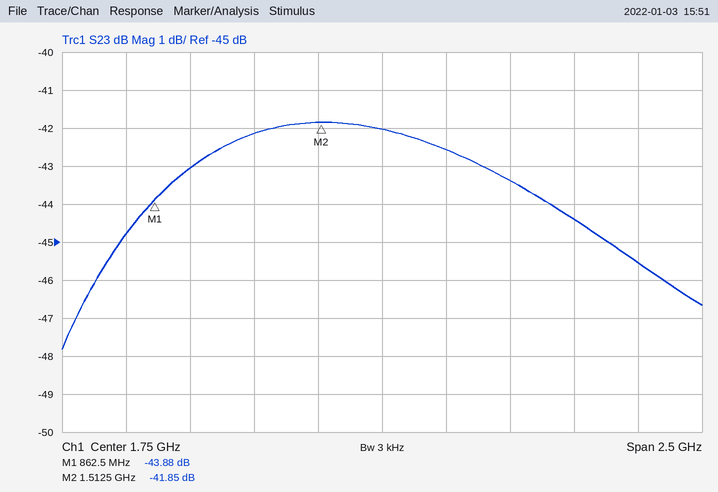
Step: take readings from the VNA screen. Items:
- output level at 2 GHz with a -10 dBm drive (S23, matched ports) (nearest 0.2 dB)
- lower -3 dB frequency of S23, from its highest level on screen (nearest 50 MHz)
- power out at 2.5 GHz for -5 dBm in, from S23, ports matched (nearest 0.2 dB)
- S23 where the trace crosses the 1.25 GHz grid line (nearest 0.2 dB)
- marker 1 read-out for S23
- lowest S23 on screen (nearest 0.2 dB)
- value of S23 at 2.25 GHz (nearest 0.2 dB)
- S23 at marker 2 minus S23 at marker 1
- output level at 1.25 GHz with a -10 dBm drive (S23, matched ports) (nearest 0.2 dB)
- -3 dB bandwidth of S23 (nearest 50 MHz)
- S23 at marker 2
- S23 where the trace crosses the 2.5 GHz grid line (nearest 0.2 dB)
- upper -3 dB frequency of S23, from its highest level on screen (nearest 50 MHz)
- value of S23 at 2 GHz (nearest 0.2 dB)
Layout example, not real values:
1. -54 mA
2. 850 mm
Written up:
1. -52.6 dBm
2. 750 MHz
3. -49.4 dBm
4. -42.2 dB
5. -43.88 dB
6. -47.8 dB
7. -43.4 dB
8. 2.03 dB
9. -52.2 dBm
10. 1.85 GHz
11. -41.85 dB
12. -44.4 dB
13. 2.60 GHz
14. -42.6 dB
